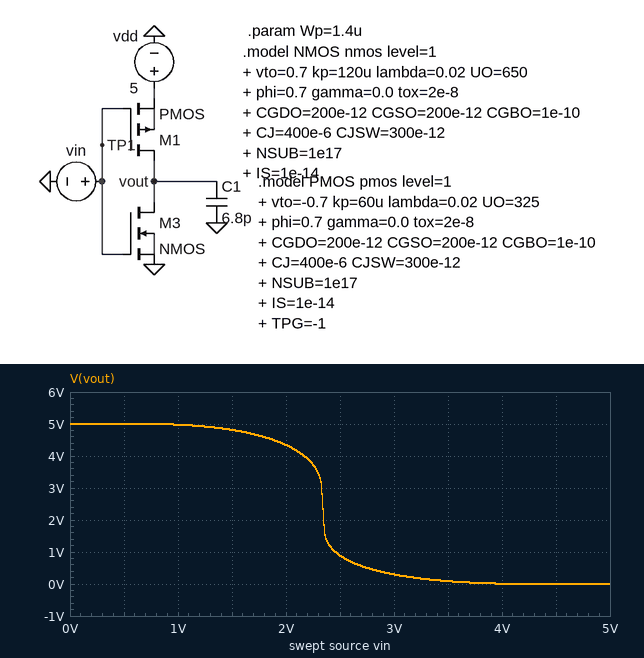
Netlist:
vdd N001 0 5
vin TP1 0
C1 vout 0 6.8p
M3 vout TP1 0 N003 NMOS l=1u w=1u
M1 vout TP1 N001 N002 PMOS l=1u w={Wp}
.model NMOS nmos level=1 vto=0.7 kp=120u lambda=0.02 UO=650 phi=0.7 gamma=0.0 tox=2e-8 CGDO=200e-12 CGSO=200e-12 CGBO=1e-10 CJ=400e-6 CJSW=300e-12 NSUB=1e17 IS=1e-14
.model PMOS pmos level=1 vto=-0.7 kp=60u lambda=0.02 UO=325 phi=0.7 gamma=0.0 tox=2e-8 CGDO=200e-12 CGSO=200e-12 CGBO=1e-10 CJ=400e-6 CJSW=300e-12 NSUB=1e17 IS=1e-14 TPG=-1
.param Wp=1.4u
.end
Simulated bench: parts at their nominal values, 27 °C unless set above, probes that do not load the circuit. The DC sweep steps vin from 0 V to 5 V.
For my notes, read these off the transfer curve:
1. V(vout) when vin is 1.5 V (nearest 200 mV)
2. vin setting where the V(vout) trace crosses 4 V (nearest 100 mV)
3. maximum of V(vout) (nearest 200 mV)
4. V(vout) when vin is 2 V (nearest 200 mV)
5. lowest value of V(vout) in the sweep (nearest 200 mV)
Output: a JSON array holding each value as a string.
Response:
["4.8 V", "2.2 V", "5.0 V", "4.4 V", "0 V"]
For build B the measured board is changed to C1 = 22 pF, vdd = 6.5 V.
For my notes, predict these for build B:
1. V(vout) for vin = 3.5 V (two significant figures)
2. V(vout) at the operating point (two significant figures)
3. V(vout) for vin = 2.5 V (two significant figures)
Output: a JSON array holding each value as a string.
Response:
["850 mV", "6.5 V", "5.6 V"]
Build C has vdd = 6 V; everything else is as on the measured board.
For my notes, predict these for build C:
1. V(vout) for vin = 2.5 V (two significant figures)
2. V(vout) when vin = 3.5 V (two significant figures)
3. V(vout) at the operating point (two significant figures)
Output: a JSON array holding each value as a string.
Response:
["4.9 V", "490 mV", "6.0 V"]
